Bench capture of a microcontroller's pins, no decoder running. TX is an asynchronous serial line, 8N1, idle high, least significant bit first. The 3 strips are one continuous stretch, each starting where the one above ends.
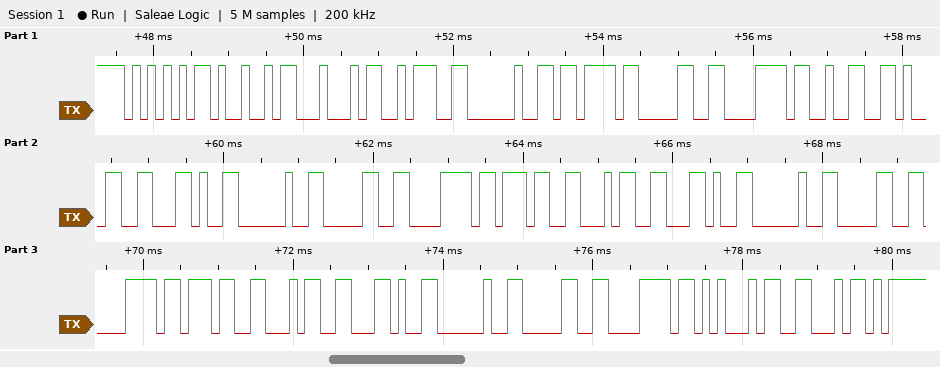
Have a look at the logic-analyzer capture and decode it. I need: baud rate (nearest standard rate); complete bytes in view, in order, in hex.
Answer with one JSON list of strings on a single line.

["9600 baud", "55 49 44 3A 20 7B 30 78 32 31 2C 20 30 78 37 34 2C 20 30 78 37 34 2C 20 30 78 45 46"]
